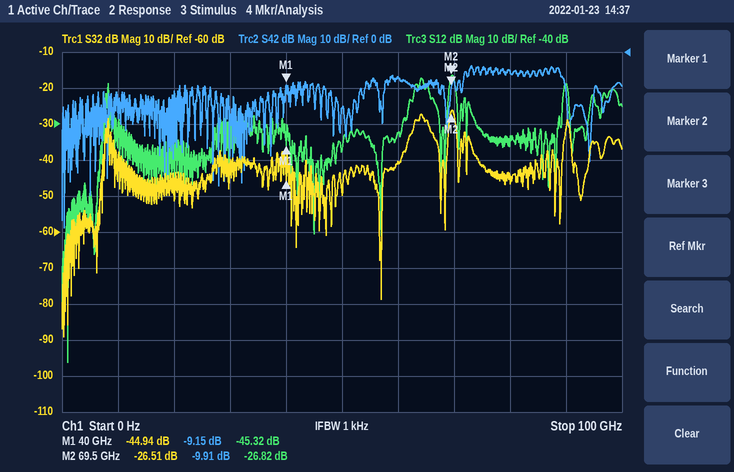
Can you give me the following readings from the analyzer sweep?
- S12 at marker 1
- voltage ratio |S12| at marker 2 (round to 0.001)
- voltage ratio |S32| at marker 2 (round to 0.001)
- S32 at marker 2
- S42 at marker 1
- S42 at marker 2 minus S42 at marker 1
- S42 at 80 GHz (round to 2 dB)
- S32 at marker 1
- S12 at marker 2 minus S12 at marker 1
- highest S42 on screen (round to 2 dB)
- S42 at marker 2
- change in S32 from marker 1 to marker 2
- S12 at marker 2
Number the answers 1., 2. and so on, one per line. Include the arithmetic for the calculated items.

1. -45.32 dB
2. 10^(-26.82/20) ≈ 0.046
3. 10^(-26.51/20) ≈ 0.047
4. -26.51 dB
5. -9.15 dB
6. -9.91 − (-9.15) = -0.76 dB
7. -6 dB
8. -44.94 dB
9. -26.82 − (-45.32) = 18.50 dB
10. -4 dB
11. -9.91 dB
12. -26.51 − (-44.94) = 18.43 dB
13. -26.82 dB
